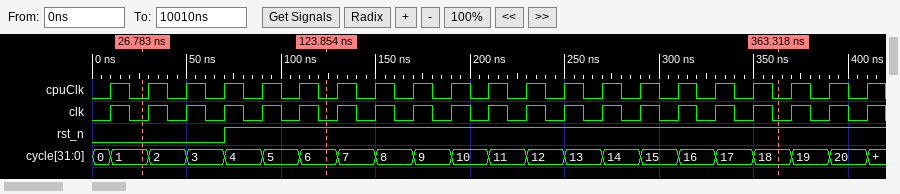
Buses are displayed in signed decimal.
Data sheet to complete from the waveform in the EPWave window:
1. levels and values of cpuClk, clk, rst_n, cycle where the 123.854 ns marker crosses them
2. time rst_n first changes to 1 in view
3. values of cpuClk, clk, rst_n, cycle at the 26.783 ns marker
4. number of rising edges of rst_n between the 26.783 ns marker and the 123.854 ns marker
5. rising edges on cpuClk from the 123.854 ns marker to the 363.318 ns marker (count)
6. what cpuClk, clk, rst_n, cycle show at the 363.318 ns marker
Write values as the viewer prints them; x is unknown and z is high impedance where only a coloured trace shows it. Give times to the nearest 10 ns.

cpuClk=0, clk=0, rst_n=1, cycle=6
70 ns
cpuClk=0, clk=0, rst_n=0, cycle=1
1
12
cpuClk=0, clk=0, rst_n=1, cycle=18
